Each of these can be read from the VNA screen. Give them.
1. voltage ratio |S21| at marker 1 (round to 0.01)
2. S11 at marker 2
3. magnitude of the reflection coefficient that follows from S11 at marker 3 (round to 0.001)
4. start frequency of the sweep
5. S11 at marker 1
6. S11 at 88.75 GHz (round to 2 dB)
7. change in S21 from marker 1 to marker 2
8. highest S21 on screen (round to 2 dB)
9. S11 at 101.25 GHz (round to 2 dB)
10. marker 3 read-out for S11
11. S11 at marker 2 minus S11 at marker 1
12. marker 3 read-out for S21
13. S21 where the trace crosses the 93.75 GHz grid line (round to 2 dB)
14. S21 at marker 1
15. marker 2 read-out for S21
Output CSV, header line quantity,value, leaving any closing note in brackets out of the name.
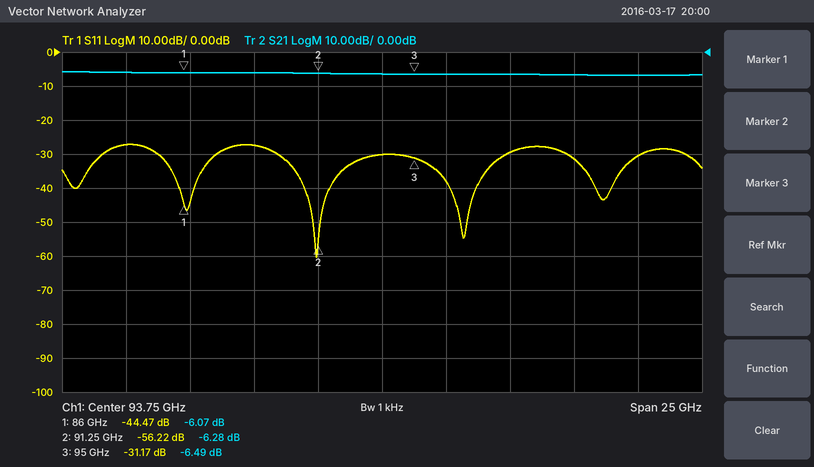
quantity,value
voltage ratio |S21| at marker 1,0.50
S11 at marker 2,-56.22 dB
magnitude of the reflection coefficient that follows from S11 at marker 3,0.028
start frequency of the sweep,81.25 GHz
S11 at marker 1,-44.47 dB
S11 at 88.75 GHz,-28 dB
change in S21 from marker 1 to marker 2,-0.21 dB
highest S21 on screen,-6 dB
S11 at 101.25 GHz,-32 dB
marker 3 read-out for S11,-31.17 dB
S11 at marker 2 minus S11 at marker 1,-11.75 dB
marker 3 read-out for S21,-6.49 dB
S21 where the trace crosses the 93.75 GHz grid line,-6 dB
S21 at marker 1,-6.07 dB
marker 2 read-out for S21,-6.28 dB
